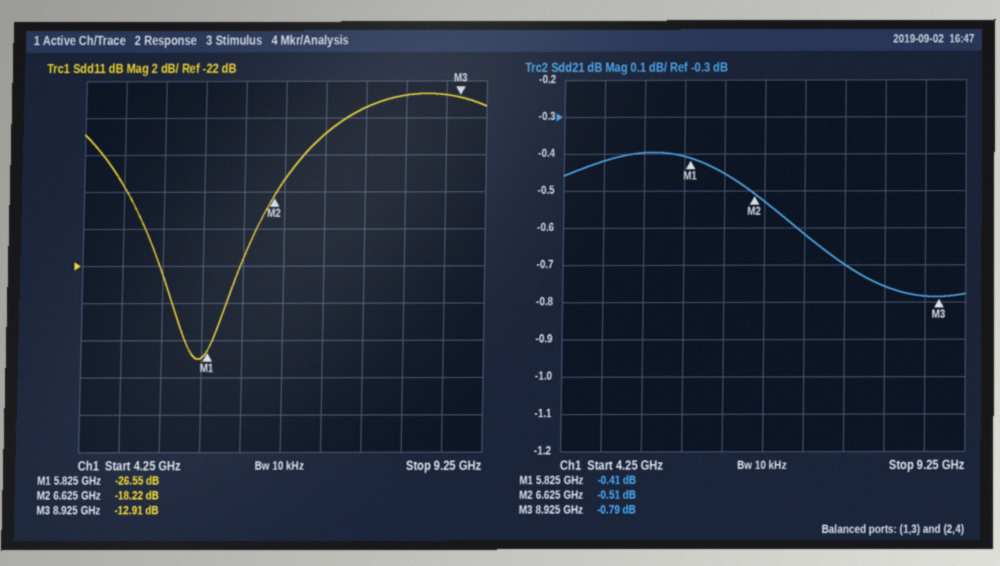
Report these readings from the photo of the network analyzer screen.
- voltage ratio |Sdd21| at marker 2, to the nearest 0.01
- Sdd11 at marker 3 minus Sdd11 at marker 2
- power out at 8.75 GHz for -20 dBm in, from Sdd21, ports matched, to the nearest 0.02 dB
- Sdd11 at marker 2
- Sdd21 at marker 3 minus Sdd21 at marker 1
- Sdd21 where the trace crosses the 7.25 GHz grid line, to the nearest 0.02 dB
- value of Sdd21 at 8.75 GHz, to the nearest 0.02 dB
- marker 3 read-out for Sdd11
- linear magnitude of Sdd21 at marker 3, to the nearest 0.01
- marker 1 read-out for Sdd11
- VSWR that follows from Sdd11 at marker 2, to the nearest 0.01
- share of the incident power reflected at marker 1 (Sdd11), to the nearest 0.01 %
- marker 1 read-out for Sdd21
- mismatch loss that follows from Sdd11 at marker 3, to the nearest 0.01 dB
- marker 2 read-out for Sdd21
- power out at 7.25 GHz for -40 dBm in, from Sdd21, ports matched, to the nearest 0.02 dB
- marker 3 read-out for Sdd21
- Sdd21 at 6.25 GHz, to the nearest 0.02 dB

0.94
5.31 dB
-20.78 dBm
-18.22 dB
-0.38 dB
-0.62 dB
-0.78 dB
-12.91 dB
0.91
-26.55 dB
1.28
0.22 %
-0.41 dB
0.23 dB
-0.51 dB
-40.62 dBm
-0.79 dB
-0.46 dB
